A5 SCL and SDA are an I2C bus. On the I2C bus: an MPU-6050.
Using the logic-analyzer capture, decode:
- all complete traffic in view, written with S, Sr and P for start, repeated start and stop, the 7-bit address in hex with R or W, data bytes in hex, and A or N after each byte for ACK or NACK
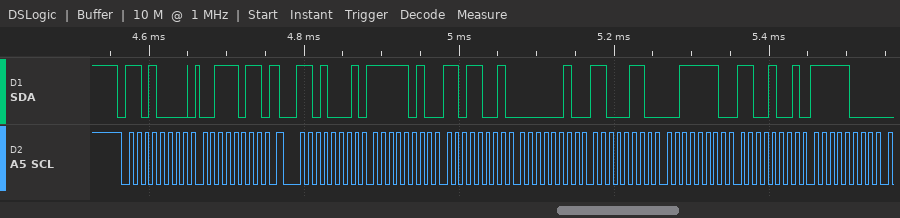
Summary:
S 68W A 3B A Sr 68R A FA A D9 A 02 A C6 A 3E A C9 A F8 A
